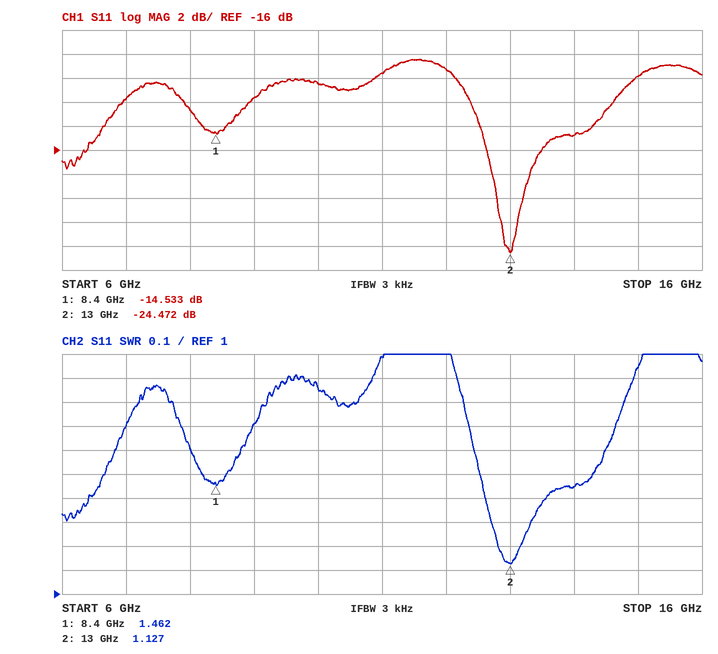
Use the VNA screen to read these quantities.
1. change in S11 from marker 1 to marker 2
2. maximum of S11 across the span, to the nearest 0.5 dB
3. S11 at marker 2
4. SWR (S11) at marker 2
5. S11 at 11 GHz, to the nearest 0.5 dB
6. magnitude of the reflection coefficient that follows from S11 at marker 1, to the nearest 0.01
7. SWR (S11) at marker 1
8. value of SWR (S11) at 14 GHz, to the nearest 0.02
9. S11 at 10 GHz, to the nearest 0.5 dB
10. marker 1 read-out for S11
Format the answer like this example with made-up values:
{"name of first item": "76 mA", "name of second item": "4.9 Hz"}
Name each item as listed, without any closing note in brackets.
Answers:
{"change in S11 from marker 1 to marker 2": "-9.939 dB", "maximum of S11 across the span, to the nearest 0.5 dB": "-8.5 dB", "S11 at marker 2": "-24.472 dB", "SWR (S11) at marker 2": "1.127", "S11 at 11 GHz, to the nearest 0.5 dB": "-9.5 dB", "magnitude of the reflection coefficient that follows from S11 at marker 1, to the nearest 0.01": "0.19", "SWR (S11) at marker 1": "1.462", "value of SWR (S11) at 14 GHz, to the nearest 0.02": "1.44", "S11 at 10 GHz, to the nearest 0.5 dB": "-10.5 dB", "marker 1 read-out for S11": "-14.533 dB"}
